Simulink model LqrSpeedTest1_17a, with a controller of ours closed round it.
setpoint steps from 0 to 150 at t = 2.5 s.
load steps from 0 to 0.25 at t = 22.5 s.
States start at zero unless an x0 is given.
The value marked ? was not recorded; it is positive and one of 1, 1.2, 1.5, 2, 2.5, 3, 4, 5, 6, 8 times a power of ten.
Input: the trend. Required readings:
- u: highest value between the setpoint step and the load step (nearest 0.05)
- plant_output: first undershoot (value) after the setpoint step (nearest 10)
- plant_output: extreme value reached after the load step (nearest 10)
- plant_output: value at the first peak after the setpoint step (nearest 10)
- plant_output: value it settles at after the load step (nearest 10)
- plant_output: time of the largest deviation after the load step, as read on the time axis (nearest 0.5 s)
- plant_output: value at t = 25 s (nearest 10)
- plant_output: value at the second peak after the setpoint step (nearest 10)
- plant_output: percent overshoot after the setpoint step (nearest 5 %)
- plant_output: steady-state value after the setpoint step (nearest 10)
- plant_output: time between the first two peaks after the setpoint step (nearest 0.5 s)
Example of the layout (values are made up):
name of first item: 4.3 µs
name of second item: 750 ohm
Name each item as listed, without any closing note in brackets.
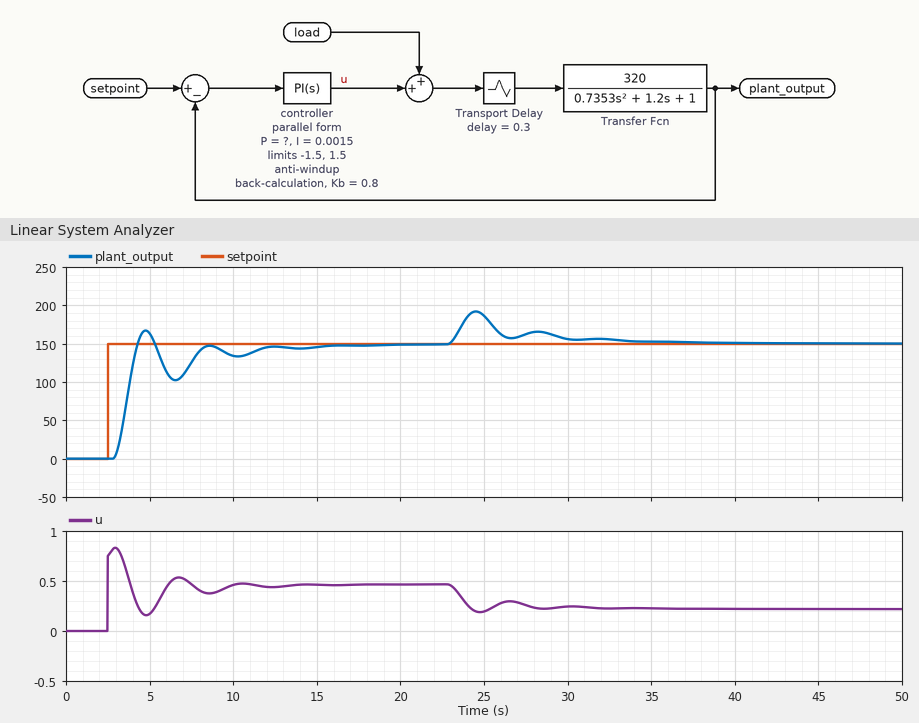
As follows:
u: highest value between the setpoint step and the load step: 0.85
plant_output: first undershoot (value) after the setpoint step: 100
plant_output: extreme value reached after the load step: 190
plant_output: value at the first peak after the setpoint step: 170
plant_output: value it settles at after the load step: 150
plant_output: time of the largest deviation after the load step, as read on the time axis: 24.5 s
plant_output: value at t = 25 s: 190
plant_output: value at the second peak after the setpoint step: 150
plant_output: percent overshoot after the setpoint step: 10 %
plant_output: steady-state value after the setpoint step: 150
plant_output: time between the first two peaks after the setpoint step: 4.0 s
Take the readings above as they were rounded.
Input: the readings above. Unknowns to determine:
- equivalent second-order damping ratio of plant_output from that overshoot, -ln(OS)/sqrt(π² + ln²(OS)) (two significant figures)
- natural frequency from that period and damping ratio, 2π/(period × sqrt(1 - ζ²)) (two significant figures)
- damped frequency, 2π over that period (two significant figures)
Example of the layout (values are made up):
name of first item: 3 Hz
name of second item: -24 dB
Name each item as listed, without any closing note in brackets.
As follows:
equivalent second-order damping ratio of plant_output from that overshoot, -ln(OS)/sqrt(π² + ln²(OS)): 0.59
natural frequency from that period and damping ratio, 2π/(period × sqrt(1 - ζ²)): 1.9 rad/s
damped frequency, 2π over that period: 1.6 rad/s
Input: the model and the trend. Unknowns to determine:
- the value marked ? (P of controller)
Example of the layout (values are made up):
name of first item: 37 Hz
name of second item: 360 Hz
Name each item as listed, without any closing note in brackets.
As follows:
the value marked ?: 0.005
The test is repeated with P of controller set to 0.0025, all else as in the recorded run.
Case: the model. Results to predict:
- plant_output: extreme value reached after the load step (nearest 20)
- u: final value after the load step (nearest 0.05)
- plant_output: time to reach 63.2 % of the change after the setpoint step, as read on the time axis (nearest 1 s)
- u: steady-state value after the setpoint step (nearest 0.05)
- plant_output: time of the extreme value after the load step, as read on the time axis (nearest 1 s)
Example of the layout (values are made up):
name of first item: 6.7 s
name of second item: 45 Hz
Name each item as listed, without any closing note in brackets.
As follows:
plant_output: extreme value reached after the load step: 200
u: final value after the load step: 0.20
plant_output: time to reach 63.2 % of the change after the setpoint step, as read on the time axis: 4 s
u: steady-state value after the setpoint step: 0.45
plant_output: time of the extreme value after the load step, as read on the time axis: 25 s
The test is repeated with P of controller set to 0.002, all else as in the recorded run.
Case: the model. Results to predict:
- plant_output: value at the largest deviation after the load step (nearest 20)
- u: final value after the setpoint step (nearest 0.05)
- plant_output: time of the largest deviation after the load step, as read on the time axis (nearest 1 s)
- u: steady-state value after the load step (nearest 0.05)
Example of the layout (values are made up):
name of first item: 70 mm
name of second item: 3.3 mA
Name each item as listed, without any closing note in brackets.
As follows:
plant_output: value at the largest deviation after the load step: 200
u: final value after the setpoint step: 0.45
plant_output: time of the largest deviation after the load step, as read on the time axis: 25 s
u: steady-state value after the load step: 0.20
